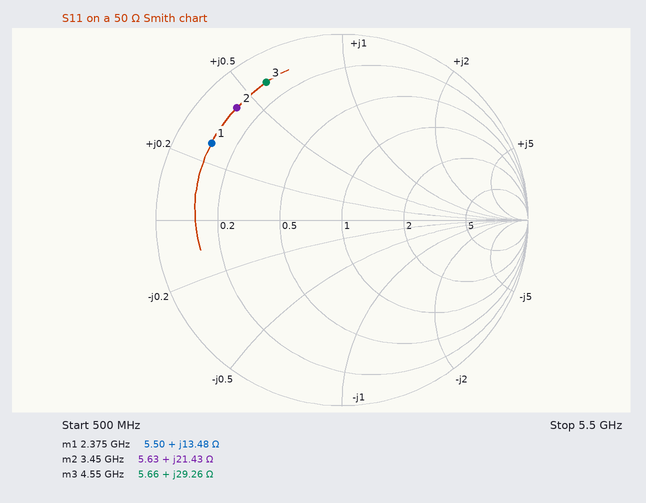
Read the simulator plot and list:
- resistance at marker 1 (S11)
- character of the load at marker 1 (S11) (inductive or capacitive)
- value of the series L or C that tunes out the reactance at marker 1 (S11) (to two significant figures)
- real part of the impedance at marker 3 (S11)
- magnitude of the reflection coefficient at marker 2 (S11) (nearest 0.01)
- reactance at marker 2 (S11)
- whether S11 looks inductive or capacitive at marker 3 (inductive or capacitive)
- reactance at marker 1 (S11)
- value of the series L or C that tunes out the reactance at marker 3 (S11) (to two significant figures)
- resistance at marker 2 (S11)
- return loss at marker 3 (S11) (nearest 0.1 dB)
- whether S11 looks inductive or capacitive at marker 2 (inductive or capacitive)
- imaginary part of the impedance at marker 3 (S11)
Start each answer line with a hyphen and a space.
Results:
- 5.50 Ω
- inductive
- 5.0 pF
- 5.66 Ω
- 0.83
- +21.43 Ω
- inductive
- +13.48 Ω
- 1.2 pF
- 5.63 Ω
- 1.5 dB
- inductive
- +29.26 Ω
